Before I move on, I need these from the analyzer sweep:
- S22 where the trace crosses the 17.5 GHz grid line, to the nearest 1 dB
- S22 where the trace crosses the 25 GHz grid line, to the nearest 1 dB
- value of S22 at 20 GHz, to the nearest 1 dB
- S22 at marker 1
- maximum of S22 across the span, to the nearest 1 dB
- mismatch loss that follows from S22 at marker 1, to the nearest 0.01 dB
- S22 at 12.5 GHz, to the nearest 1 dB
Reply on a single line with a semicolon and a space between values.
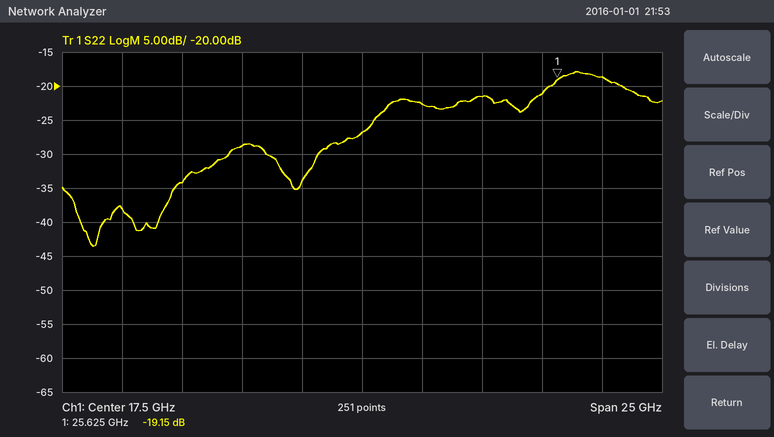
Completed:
-27 dB; -21 dB; -23 dB; -19.15 dB; -18 dB; 0.05 dB; -29 dB
